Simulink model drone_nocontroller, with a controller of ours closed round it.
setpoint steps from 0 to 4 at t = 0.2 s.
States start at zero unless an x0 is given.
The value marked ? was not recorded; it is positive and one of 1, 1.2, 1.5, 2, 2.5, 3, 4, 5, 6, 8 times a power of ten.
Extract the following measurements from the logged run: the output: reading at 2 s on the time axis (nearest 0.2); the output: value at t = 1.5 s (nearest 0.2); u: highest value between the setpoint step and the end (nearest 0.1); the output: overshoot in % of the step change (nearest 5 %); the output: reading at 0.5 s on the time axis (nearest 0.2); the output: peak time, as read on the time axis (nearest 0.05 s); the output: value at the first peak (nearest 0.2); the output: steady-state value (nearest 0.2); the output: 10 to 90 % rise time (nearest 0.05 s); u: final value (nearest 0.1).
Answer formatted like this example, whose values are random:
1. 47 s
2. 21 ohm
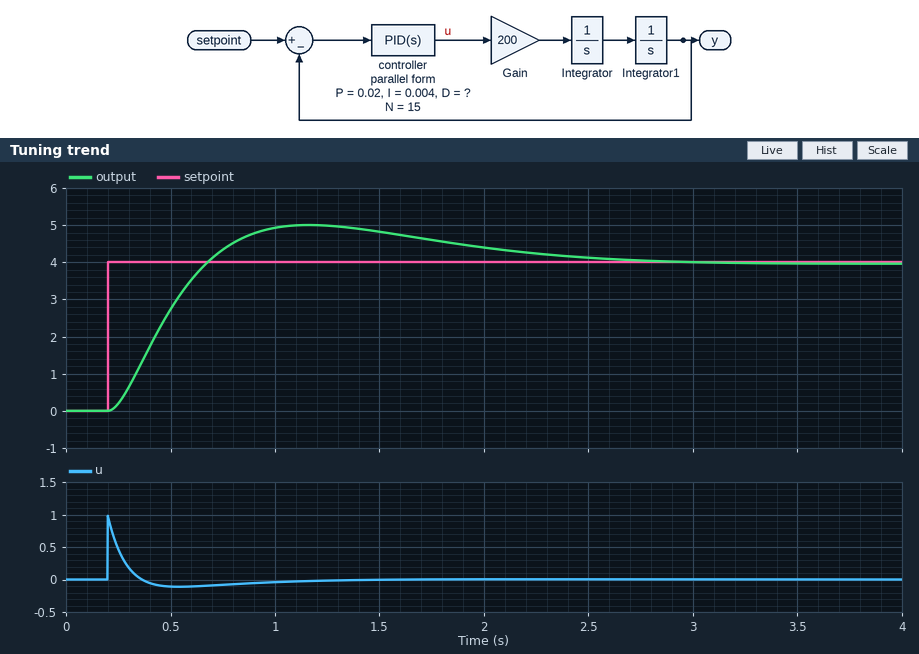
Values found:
1. 4.4
2. 4.8
3. 1.0
4. 25 %
5. 2.8
6. 1.15 s
7. 5.0
8. 4.0
9. 0.35 s
10. 0.0
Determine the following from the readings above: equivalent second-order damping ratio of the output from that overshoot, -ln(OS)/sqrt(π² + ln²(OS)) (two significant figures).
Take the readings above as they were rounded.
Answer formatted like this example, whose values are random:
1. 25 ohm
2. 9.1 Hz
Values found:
1. 0.40
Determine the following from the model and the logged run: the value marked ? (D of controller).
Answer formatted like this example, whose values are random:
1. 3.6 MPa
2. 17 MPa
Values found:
1. 0.015
